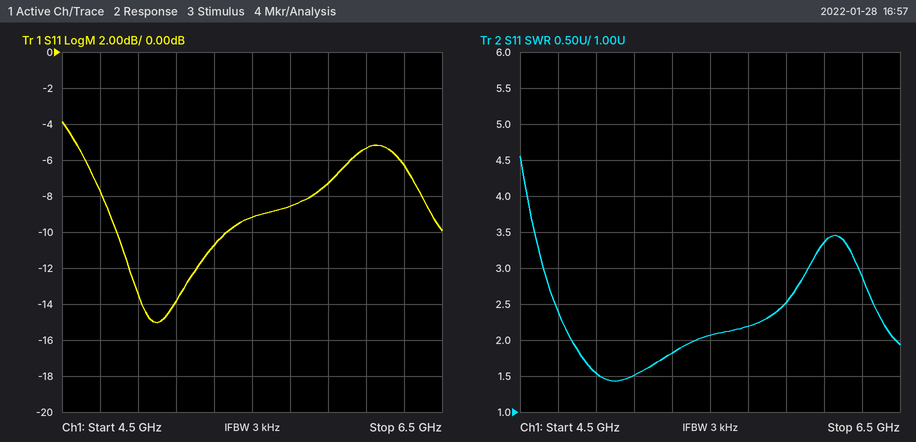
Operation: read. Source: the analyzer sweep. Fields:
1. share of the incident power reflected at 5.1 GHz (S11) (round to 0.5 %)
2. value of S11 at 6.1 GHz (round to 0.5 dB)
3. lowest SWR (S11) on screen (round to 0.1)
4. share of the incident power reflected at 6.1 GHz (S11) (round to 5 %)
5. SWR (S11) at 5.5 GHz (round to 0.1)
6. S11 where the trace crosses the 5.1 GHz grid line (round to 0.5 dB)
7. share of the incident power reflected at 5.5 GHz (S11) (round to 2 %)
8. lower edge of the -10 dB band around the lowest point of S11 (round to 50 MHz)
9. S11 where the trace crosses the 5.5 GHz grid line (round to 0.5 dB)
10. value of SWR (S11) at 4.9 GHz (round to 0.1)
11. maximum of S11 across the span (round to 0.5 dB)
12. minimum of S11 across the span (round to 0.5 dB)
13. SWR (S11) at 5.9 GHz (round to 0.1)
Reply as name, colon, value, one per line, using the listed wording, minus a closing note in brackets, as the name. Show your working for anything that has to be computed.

share of the incident power reflected at 5.1 GHz (S11): 10^(-14/10) ≈ 4.0 %
value of S11 at 6.1 GHz: -5.5 dB
lowest SWR (S11) on screen: 1.4
share of the incident power reflected at 6.1 GHz (S11): 10^(-5.5/10) ≈ 28.2 %, so 30 % to the nearest 5 %
SWR (S11) at 5.5 GHz: 2.1
S11 where the trace crosses the 5.1 GHz grid line: -14.0 dB
share of the incident power reflected at 5.5 GHz (S11): 10^(-9/10) ≈ 12.6 %, so 12 % to the nearest 2 %
lower edge of the -10 dB band around the lowest point of S11: 4.80 GHz
S11 where the trace crosses the 5.5 GHz grid line: -9.0 dB
value of SWR (S11) at 4.9 GHz: 1.5
maximum of S11 across the span: -4.0 dB
minimum of S11 across the span: -15.0 dB
SWR (S11) at 5.9 GHz: 2.5
